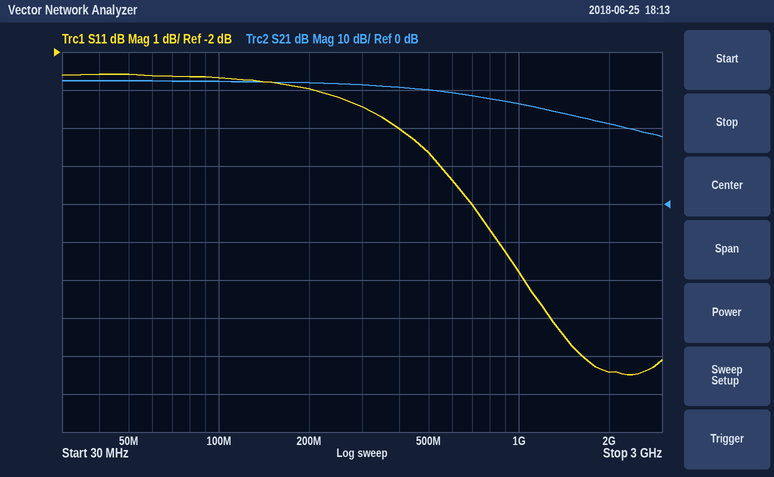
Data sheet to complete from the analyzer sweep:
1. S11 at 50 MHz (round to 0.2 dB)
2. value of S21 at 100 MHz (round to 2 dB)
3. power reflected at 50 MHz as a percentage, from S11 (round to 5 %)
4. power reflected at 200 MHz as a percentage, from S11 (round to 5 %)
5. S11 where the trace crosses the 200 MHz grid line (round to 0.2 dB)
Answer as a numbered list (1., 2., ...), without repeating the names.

1. -2.6 dB
2. 32 dB
3. 55 %
4. 50 %
5. -3.0 dB
